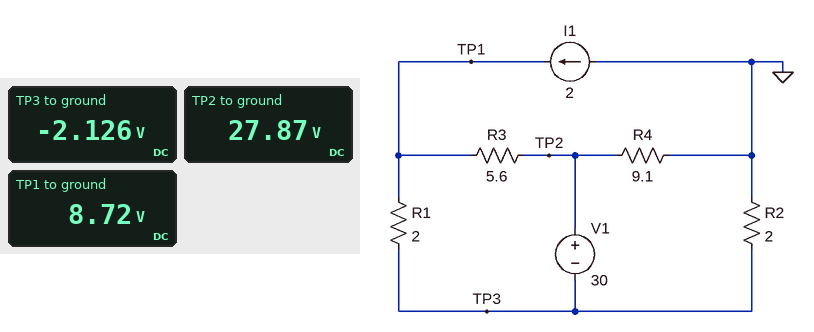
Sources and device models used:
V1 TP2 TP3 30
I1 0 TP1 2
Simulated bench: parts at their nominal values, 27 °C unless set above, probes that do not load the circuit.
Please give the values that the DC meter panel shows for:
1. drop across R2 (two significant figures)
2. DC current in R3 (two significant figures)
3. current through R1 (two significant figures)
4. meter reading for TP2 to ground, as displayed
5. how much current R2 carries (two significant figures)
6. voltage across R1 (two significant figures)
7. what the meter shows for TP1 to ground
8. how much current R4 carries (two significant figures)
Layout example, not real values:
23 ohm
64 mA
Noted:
2.1 V
3.4 A
5.4 A
27.87 V
1.1 A
11 V
8.72 V
3.1 A
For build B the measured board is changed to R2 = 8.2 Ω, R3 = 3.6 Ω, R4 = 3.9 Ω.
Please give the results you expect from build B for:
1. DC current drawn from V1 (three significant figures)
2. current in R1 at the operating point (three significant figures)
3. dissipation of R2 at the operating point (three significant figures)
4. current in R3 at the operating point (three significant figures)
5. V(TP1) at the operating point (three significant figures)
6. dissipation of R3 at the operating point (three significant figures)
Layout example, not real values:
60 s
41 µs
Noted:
8.48 A
6.64 A
27.6 W
4.64 A
-1.76 V
77.6 W
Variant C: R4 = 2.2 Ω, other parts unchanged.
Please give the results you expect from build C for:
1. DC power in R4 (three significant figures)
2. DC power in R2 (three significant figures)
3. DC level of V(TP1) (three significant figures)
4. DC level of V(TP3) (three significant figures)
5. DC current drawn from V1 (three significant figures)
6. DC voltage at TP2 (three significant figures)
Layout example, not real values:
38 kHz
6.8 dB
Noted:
144 W
74.3 W
-1.35 V
-12.2 V
11.5 A
17.8 V
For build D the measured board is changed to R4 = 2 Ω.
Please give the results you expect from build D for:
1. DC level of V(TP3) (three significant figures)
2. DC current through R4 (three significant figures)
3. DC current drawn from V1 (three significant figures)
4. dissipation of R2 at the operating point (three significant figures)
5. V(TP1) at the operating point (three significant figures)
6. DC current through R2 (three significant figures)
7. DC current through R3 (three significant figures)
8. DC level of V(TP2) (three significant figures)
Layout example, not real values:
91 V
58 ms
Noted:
-13.0 V
8.50 A
11.9 A
84.5 W
-2.16 V
6.50 A
3.42 A
17.0 V
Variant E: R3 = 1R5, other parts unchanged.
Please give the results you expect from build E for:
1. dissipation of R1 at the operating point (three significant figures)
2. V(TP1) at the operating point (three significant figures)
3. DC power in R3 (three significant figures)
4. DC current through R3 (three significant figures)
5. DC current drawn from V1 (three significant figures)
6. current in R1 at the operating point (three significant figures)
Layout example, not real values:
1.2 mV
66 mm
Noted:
178 W
16.7 V
82.8 W
7.43 A
10.5 A
9.43 A
